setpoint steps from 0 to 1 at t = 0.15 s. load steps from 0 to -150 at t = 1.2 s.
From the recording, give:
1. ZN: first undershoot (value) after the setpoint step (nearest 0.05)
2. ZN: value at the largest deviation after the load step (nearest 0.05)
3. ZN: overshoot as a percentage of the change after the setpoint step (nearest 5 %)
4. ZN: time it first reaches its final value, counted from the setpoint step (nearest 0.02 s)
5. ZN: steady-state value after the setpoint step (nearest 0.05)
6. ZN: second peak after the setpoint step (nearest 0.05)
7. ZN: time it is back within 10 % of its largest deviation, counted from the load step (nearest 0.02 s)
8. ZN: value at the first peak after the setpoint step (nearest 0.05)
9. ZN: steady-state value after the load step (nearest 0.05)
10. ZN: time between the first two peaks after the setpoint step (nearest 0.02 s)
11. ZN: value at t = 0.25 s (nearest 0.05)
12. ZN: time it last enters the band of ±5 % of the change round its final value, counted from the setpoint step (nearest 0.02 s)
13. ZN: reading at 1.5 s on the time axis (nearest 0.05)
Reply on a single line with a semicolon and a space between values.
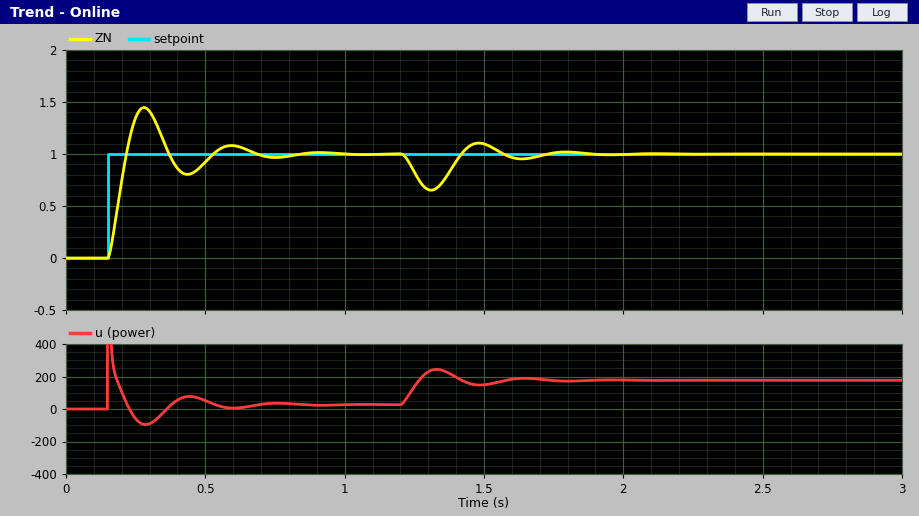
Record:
0.80; 0.65; 45 %; 0.06 s; 1.00; 1.10; 0.48 s; 1.45; 1.00; 0.32 s; 1.35; 0.50 s; 1.10
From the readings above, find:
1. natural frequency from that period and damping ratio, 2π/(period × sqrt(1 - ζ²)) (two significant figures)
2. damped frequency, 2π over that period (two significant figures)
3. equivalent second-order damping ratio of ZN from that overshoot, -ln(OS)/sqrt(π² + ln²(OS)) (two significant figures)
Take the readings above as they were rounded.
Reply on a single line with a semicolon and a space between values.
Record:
20 rad/s; 20 rad/s; 0.25
